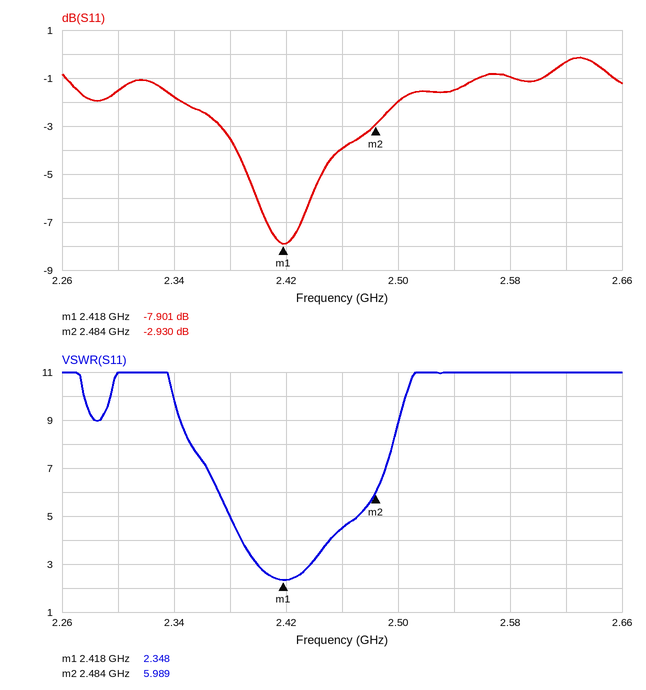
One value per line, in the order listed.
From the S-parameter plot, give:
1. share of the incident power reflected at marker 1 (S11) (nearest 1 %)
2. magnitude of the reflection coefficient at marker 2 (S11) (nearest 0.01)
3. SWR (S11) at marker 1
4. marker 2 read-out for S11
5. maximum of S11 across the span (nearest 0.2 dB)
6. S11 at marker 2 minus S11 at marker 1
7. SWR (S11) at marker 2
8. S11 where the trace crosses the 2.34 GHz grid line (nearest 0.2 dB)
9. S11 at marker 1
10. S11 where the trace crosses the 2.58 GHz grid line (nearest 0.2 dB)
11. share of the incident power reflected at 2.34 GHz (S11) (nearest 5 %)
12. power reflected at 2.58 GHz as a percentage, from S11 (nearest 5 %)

16 %
0.71
2.348
-2.930 dB
-0.2 dB
4.971 dB
5.989
-1.8 dB
-7.901 dB
-1.0 dB
65 %
80 %
